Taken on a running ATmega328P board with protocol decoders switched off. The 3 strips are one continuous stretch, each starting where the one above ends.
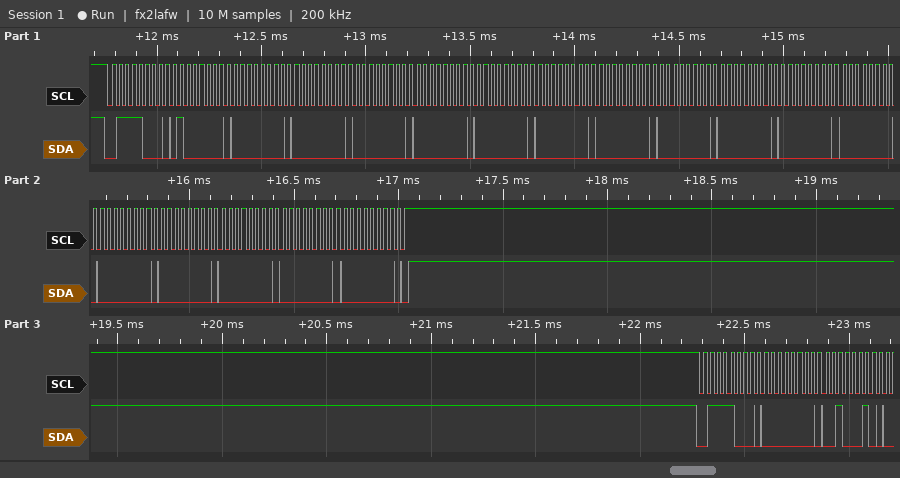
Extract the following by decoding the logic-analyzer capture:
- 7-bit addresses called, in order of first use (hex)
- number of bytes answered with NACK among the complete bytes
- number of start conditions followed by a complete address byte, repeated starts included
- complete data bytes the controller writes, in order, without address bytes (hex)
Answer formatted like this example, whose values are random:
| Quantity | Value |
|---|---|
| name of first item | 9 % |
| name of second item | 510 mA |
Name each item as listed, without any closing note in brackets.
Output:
| Quantity | Value |
|---|---|
| 7-bit addresses called, in order of first use | 0x3C |
| number of bytes answered with NACK among the complete bytes | 0 |
| number of start conditions followed by a complete address byte, repeated starts included | 2 |
| complete data bytes the controller writes, in order, without address bytes | 40 00 00 00 00 00 00 00 00 00 00 00 00 00 00 00 00 00 22 |
